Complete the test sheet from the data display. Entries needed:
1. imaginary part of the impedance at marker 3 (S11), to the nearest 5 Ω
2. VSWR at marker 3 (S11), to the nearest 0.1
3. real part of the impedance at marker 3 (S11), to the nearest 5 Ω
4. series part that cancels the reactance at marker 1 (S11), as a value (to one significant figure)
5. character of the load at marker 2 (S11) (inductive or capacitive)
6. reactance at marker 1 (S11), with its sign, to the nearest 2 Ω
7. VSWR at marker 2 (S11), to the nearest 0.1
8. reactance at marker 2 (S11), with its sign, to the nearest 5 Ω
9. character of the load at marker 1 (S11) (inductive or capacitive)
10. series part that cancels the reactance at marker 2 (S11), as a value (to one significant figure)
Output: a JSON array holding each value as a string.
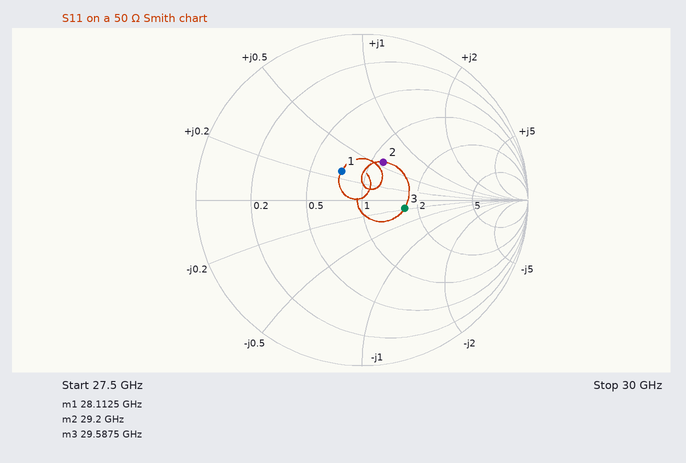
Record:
["-10 Ω", "1.7", "85 Ω", "400 fF", "inductive", "+14 Ω", "1.7", "+30 Ω", "inductive", "200 fF"]
